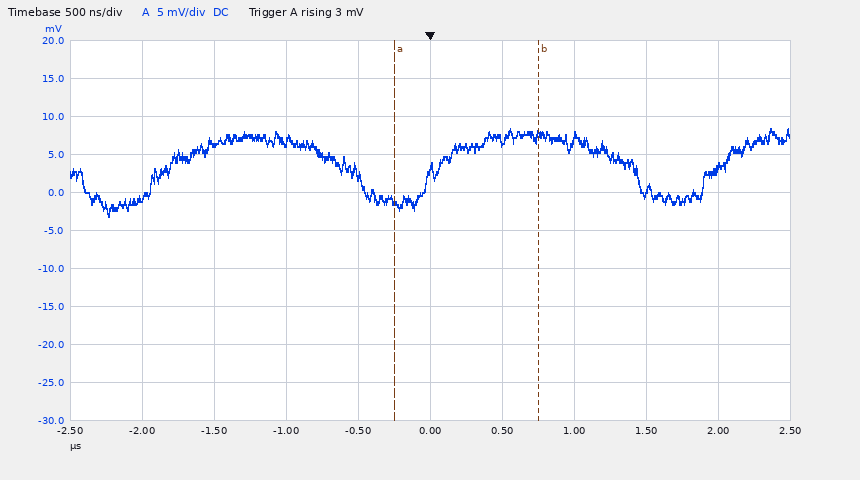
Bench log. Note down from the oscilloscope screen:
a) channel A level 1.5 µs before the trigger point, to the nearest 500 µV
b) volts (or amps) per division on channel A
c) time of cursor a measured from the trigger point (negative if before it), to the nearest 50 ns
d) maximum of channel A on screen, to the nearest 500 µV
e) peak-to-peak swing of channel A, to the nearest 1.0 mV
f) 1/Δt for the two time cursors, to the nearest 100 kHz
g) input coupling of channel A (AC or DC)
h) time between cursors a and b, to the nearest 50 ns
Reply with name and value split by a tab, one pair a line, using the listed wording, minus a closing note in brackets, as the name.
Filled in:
channel A level 1.5 µs before the trigger point, to the nearest 500 µV	6.5 mV
volts (or amps) per division on channel A	5 mV
time of cursor a measured from the trigger point (negative if before it), to the nearest 50 ns	-250 ns
maximum of channel A on screen, to the nearest 500 µV	8.5 mV
peak-to-peak swing of channel A, to the nearest 1.0 mV	12.0 mV
1/Δt for the two time cursors, to the nearest 100 kHz	1.0 MHz
input coupling of channel A	DC
time between cursors a and b, to the nearest 50 ns	1.00 µs
